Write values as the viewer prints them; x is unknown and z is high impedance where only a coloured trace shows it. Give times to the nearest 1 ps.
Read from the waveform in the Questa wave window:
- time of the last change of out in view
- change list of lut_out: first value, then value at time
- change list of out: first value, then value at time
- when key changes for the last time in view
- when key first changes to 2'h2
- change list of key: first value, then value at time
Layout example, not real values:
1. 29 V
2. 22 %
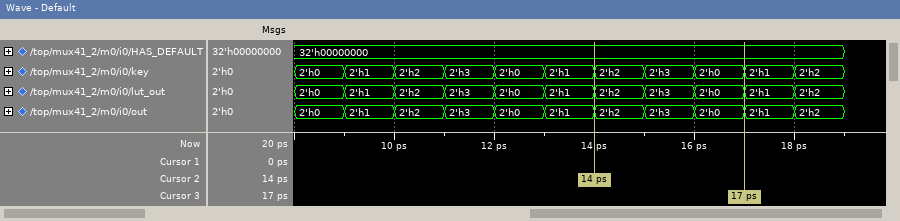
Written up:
1. 18 ps
2. 2'h0, 2'h1 at 9 ps, 2'h2 at 10 ps, 2'h3 at 11 ps, 2'h0 at 12 ps, 2'h1 at 13 ps, 2'h2 at 14 ps, 2'h3 at 15 ps, 2'h0 at 16 ps, 2'h1 at 17 ps, 2'h2 at 18 ps
3. 2'h0, 2'h1 at 9 ps, 2'h2 at 10 ps, 2'h3 at 11 ps, 2'h0 at 12 ps, 2'h1 at 13 ps, 2'h2 at 14 ps, 2'h3 at 15 ps, 2'h0 at 16 ps, 2'h1 at 17 ps, 2'h2 at 18 ps
4. 18 ps
5. 10 ps
6. 2'h0, 2'h1 at 9 ps, 2'h2 at 10 ps, 2'h3 at 11 ps, 2'h0 at 12 ps, 2'h1 at 13 ps, 2'h2 at 14 ps, 2'h3 at 15 ps, 2'h0 at 16 ps, 2'h1 at 17 ps, 2'h2 at 18 ps
